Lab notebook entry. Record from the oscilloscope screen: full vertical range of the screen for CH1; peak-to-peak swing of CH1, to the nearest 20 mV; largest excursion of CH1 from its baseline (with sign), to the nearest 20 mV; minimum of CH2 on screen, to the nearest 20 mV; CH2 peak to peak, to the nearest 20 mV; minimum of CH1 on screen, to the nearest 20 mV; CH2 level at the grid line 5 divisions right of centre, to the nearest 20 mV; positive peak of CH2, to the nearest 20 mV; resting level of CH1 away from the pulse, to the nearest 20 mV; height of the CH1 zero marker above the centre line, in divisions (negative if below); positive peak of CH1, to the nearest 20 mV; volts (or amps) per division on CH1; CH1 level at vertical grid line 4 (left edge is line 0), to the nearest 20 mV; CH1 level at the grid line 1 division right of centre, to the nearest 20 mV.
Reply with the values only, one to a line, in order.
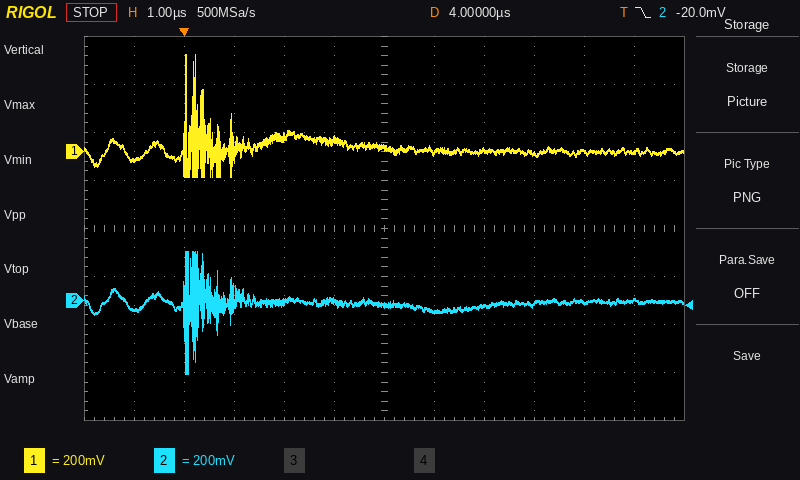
1.6 V
500 mV
+400 mV
-300 mV
500 mV
-100 mV
0 mV
200 mV
0 mV
+1.6 div
400 mV
200 mV
60 mV
0 mV
